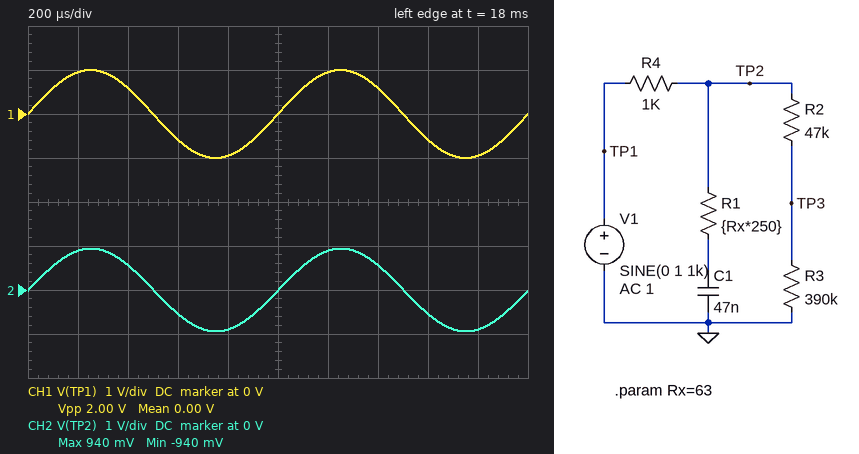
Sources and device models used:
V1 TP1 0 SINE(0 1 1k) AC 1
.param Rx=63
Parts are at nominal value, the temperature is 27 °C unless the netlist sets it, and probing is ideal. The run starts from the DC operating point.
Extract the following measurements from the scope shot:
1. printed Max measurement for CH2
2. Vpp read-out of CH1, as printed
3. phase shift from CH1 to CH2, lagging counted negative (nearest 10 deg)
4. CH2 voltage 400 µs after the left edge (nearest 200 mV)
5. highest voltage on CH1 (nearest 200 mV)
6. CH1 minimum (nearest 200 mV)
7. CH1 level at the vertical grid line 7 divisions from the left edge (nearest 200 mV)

940 mV
2.00 V
0 deg
600 mV
1.0 V
-1.0 V
600 mV
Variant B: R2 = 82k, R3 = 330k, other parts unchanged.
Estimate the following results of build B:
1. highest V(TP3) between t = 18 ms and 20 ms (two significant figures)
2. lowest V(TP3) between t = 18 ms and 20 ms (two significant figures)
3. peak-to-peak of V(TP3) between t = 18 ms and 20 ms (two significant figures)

750 mV
-750 mV
1.5 V
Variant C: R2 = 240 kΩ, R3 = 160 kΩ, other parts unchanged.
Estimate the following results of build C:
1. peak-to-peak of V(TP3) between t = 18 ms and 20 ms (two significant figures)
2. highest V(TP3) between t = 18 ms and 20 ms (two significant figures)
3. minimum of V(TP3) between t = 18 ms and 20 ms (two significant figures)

750 mV
380 mV
-380 mV
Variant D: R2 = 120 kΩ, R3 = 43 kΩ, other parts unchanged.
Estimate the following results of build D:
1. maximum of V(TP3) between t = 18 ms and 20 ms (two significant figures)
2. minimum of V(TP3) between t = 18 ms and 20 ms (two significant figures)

250 mV
-250 mV
